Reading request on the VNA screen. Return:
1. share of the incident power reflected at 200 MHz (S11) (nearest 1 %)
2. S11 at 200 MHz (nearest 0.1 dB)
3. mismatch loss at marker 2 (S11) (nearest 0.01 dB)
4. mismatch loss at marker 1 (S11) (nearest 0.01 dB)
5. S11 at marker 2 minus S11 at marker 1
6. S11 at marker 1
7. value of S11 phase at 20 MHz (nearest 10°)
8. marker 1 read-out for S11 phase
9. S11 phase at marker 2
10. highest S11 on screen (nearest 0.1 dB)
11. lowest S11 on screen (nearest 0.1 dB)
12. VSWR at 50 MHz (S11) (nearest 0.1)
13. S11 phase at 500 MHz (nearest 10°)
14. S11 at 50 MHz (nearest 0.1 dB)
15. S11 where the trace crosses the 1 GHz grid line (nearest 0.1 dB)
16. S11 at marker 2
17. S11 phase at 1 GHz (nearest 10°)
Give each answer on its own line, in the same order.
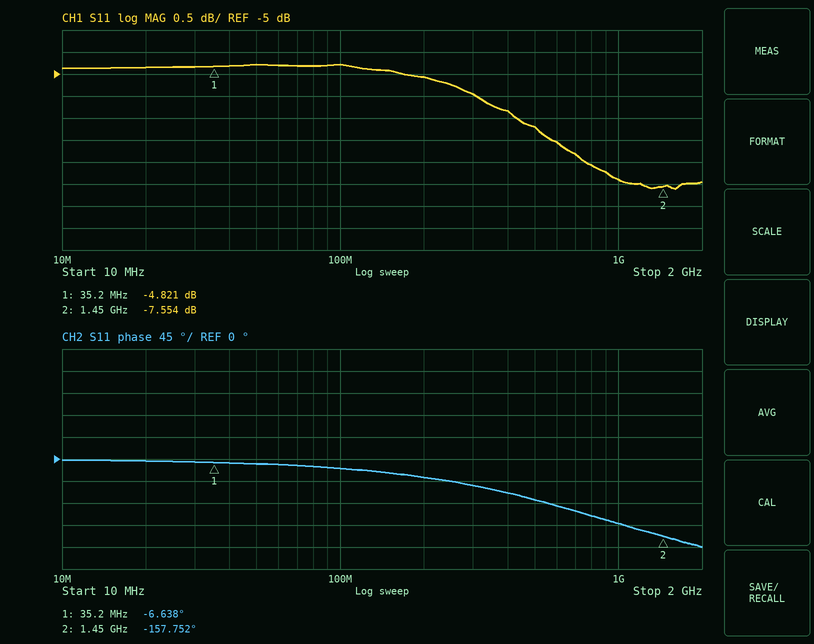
31 %
-5.1 dB
0.84 dB
1.74 dB
-2.733 dB
-4.821 dB
0°
-6.638°
-157.752°
-4.8 dB
-7.6 dB
3.7
-80°
-4.8 dB
-7.4 dB
-7.554 dB
-130°
